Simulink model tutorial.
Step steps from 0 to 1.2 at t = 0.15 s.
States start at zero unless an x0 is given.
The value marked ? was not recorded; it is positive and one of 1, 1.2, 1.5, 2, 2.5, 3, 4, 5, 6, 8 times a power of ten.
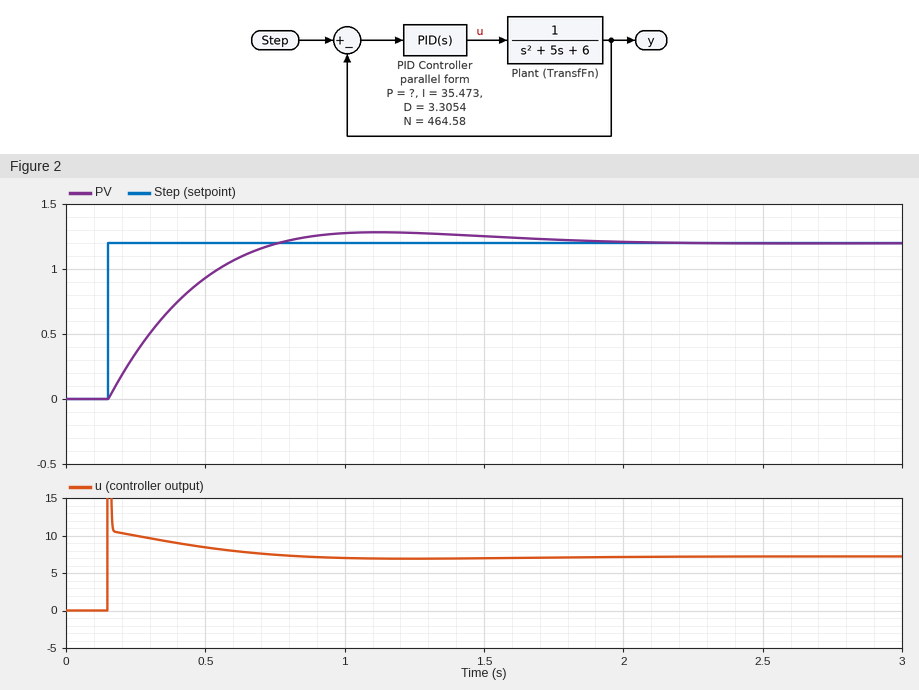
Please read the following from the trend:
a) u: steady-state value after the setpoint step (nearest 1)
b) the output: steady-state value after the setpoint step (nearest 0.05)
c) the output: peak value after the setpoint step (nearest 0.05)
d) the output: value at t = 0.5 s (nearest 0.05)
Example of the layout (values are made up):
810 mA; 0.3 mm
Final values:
7; 1.20; 1.30; 0.95
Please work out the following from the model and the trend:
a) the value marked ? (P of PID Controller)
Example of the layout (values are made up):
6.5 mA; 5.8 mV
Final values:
20
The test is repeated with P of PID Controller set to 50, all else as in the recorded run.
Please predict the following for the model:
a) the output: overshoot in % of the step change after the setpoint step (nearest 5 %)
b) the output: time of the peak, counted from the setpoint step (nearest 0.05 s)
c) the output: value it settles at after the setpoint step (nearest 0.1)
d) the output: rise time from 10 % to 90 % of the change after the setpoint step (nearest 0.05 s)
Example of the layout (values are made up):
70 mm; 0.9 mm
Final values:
10 %; 0.45 s; 1.2; 0.20 s
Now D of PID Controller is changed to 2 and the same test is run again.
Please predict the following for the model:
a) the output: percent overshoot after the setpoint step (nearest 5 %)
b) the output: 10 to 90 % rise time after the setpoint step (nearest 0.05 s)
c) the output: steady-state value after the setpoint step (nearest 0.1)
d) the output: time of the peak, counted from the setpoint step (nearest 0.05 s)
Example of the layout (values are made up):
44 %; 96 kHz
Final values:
10 %; 0.40 s; 1.2; 0.85 s
